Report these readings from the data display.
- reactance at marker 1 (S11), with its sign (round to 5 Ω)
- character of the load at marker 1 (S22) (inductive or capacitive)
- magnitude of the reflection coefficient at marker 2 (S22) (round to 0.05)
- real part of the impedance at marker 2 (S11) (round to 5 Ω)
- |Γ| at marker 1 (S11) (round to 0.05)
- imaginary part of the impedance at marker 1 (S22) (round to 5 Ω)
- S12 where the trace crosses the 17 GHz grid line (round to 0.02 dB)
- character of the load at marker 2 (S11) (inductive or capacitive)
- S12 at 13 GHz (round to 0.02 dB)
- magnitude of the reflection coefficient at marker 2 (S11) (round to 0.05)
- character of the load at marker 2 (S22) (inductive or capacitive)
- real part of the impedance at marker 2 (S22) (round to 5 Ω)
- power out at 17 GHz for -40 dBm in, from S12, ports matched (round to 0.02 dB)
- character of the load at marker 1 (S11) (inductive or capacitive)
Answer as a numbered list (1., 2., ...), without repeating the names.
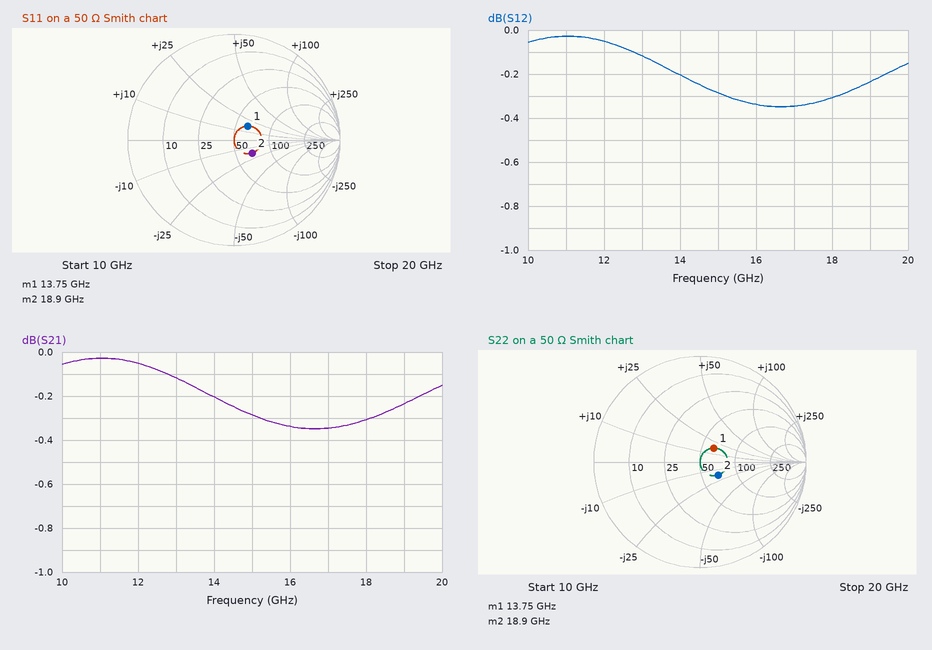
1. +15 Ω
2. inductive
3. 0.20
4. 70 Ω
5. 0.20
6. +15 Ω
7. -0.34 dB
8. capacitive
9. -0.12 dB
10. 0.20
11. capacitive
12. 70 Ω
13. -40.34 dBm
14. inductive
